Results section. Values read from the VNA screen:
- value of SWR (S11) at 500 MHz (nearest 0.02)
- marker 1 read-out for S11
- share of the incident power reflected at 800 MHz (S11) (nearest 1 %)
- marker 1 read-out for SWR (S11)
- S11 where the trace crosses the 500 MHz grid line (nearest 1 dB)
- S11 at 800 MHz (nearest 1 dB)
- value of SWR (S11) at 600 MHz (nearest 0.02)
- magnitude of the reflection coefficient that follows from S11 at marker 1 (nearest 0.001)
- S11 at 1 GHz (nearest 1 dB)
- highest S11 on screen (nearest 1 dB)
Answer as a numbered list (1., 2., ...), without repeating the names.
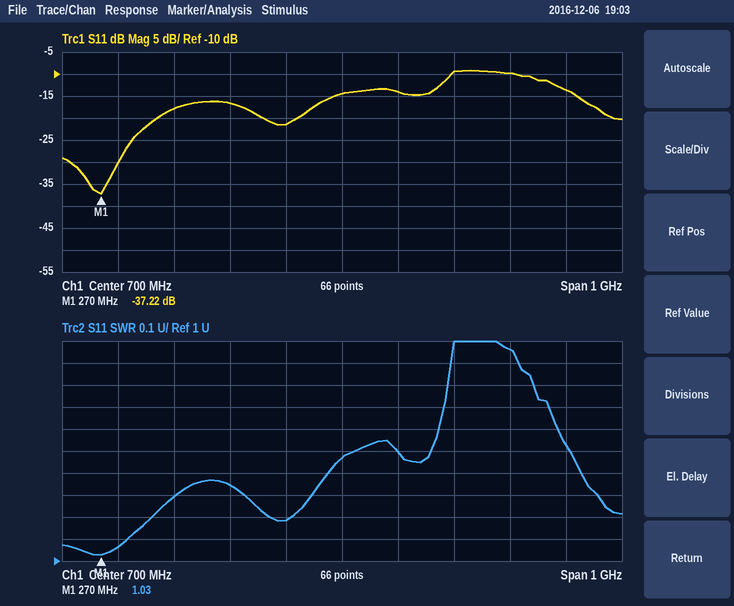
1. 1.34
2. -37.22 dB
3. 4 %
4. 1.03
5. -17 dB
6. -14 dB
7. 1.18
8. 0.014
9. -10 dB
10. -9 dB
